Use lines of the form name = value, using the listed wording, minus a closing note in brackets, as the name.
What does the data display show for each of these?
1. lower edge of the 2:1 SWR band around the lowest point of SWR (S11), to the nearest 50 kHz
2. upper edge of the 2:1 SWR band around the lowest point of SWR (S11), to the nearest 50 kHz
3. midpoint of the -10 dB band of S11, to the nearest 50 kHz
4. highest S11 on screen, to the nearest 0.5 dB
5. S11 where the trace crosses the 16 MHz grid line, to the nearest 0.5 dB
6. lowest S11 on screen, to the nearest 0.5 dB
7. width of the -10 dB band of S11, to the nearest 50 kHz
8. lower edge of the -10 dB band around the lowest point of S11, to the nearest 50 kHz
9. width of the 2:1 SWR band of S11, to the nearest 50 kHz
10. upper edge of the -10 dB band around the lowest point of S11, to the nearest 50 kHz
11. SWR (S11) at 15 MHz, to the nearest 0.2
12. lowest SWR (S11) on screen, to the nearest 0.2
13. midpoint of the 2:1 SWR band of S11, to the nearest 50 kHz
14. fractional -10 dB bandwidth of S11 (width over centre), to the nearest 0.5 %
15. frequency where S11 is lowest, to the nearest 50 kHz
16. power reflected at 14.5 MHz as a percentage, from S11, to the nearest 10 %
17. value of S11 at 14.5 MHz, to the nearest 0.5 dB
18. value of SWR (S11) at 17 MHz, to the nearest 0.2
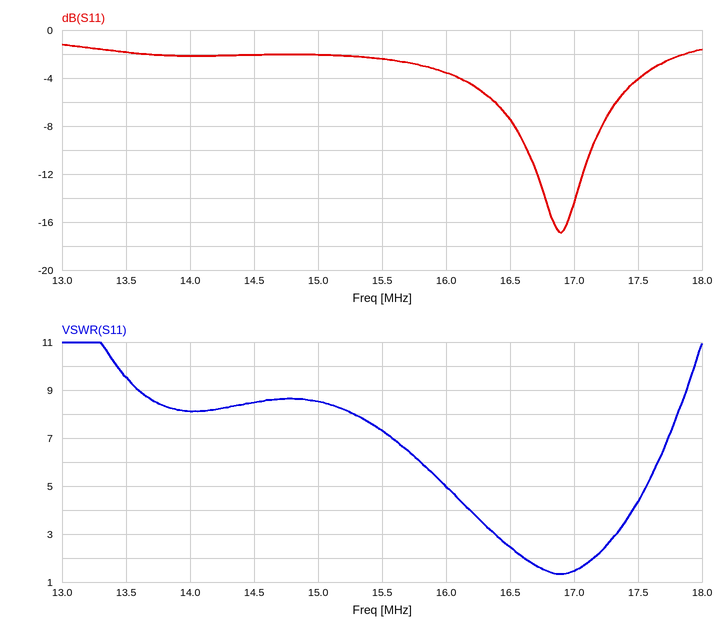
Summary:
lower edge of the 2:1 SWR band around the lowest point of SWR (S11), to the nearest 50 kHz = 16.60 MHz
upper edge of the 2:1 SWR band around the lowest point of SWR (S11), to the nearest 50 kHz = 17.15 MHz
midpoint of the -10 dB band of S11, to the nearest 50 kHz = 16.90 MHz
highest S11 on screen, to the nearest 0.5 dB = -1.0 dB
S11 where the trace crosses the 16 MHz grid line, to the nearest 0.5 dB = -3.5 dB
lowest S11 on screen, to the nearest 0.5 dB = -17.0 dB
width of the -10 dB band of S11, to the nearest 50 kHz = 500 kHz
lower edge of the -10 dB band around the lowest point of S11, to the nearest 50 kHz = 16.65 MHz
width of the 2:1 SWR band of S11, to the nearest 50 kHz = 550 kHz
upper edge of the -10 dB band around the lowest point of S11, to the nearest 50 kHz = 17.15 MHz
SWR (S11) at 15 MHz, to the nearest 0.2 = 8.6
lowest SWR (S11) on screen, to the nearest 0.2 = 1.4
midpoint of the 2:1 SWR band of S11, to the nearest 50 kHz = 16.90 MHz
fractional -10 dB bandwidth of S11 (width over centre), to the nearest 0.5 % = 3.0 %
frequency where S11 is lowest, to the nearest 50 kHz = 16.90 MHz
power reflected at 14.5 MHz as a percentage, from S11, to the nearest 10 % = 60 %
value of S11 at 14.5 MHz, to the nearest 0.5 dB = -2.0 dB
value of SWR (S11) at 17 MHz, to the nearest 0.2 = 1.4
